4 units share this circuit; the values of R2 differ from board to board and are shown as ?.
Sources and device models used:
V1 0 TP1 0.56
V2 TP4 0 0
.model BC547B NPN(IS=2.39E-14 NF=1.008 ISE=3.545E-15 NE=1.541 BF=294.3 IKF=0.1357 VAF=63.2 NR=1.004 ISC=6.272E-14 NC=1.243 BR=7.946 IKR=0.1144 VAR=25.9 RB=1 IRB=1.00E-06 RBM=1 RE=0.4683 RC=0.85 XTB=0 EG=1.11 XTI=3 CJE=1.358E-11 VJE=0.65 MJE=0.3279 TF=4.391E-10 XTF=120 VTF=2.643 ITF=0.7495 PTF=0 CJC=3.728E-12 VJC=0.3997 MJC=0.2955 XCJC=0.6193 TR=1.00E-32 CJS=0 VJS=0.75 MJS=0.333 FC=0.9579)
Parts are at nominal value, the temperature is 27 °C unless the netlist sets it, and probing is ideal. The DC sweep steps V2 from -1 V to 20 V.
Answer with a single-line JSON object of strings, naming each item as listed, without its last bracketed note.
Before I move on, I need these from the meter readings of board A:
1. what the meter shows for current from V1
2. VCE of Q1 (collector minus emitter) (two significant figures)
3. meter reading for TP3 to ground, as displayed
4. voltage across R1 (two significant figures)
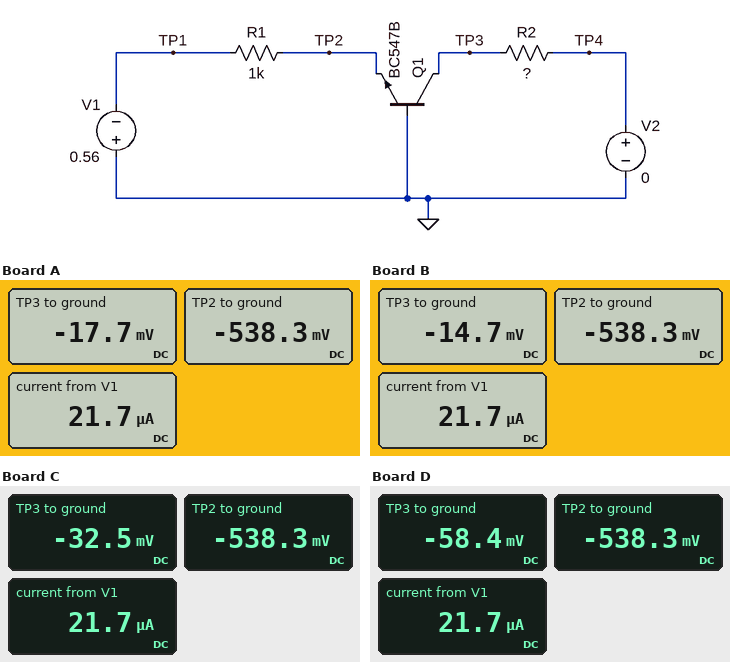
{"what the meter shows for current from V1": "21.7 µA", "VCE of Q1 (collector minus emitter)": "520 mV", "meter reading for TP3 to ground, as displayed": "-17.7 mV", "voltage across R1": "22 mV"}
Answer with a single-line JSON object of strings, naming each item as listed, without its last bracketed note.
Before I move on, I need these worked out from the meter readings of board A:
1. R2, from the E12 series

{"R2, from the E12 series": "820 Ω"}
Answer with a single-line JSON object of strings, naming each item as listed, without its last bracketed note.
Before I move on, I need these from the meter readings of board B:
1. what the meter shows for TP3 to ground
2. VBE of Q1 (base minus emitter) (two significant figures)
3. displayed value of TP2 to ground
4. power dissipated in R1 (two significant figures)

{"what the meter shows for TP3 to ground": "-14.7 mV", "VBE of Q1 (base minus emitter)": "540 mV", "displayed value of TP2 to ground": "-538.3 mV", "power dissipated in R1": "470 nW"}
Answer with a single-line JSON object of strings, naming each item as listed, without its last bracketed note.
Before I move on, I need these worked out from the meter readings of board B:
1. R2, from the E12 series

{"R2, from the E12 series": "680 Ω"}
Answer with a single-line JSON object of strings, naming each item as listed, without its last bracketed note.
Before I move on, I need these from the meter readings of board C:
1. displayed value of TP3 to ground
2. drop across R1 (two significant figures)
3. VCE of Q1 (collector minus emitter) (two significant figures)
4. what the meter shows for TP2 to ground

{"displayed value of TP3 to ground": "-32.5 mV", "drop across R1": "22 mV", "VCE of Q1 (collector minus emitter)": "510 mV", "what the meter shows for TP2 to ground": "-538.3 mV"}
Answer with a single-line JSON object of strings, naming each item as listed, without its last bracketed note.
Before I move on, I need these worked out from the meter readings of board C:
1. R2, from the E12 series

{"R2, from the E12 series": "1.5 kΩ"}
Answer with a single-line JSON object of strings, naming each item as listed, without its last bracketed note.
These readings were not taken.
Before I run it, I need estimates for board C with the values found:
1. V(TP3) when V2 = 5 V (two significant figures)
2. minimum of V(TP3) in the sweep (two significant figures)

{"V(TP3) when V2 = 5 V": "5.0 V", "minimum of V(TP3) in the sweep": "-640 mV"}
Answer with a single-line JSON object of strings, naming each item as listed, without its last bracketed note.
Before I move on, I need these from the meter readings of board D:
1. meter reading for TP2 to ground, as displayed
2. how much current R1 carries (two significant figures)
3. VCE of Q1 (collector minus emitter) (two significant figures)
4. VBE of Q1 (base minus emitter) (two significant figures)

{"meter reading for TP2 to ground, as displayed": "-538.3 mV", "how much current R1 carries": "22 µA", "VCE of Q1 (collector minus emitter)": "480 mV", "VBE of Q1 (base minus emitter)": "540 mV"}
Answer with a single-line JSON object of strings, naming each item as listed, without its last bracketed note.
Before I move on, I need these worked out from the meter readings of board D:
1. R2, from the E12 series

{"R2, from the E12 series": "2.7 kΩ"}
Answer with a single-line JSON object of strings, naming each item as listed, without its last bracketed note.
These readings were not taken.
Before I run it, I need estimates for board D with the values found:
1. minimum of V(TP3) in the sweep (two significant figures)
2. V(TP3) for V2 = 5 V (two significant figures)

{"minimum of V(TP3) in the sweep": "-620 mV", "V(TP3) for V2 = 5 V": "4.9 V"}
